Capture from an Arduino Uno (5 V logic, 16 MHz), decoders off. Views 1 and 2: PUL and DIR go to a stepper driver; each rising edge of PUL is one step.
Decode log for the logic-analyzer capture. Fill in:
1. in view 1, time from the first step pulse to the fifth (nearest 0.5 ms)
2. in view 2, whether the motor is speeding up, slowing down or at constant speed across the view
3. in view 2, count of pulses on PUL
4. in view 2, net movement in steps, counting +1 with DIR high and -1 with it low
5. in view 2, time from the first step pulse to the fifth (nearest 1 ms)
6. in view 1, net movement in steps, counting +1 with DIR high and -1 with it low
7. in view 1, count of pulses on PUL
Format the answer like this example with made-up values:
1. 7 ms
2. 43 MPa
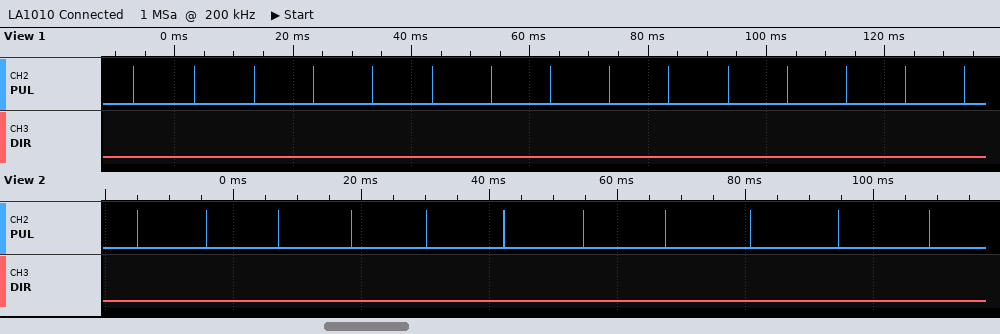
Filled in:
1. 40.5 ms
2. slowing down
3. 11
4. -11
5. 45 ms
6. -15
7. 15
